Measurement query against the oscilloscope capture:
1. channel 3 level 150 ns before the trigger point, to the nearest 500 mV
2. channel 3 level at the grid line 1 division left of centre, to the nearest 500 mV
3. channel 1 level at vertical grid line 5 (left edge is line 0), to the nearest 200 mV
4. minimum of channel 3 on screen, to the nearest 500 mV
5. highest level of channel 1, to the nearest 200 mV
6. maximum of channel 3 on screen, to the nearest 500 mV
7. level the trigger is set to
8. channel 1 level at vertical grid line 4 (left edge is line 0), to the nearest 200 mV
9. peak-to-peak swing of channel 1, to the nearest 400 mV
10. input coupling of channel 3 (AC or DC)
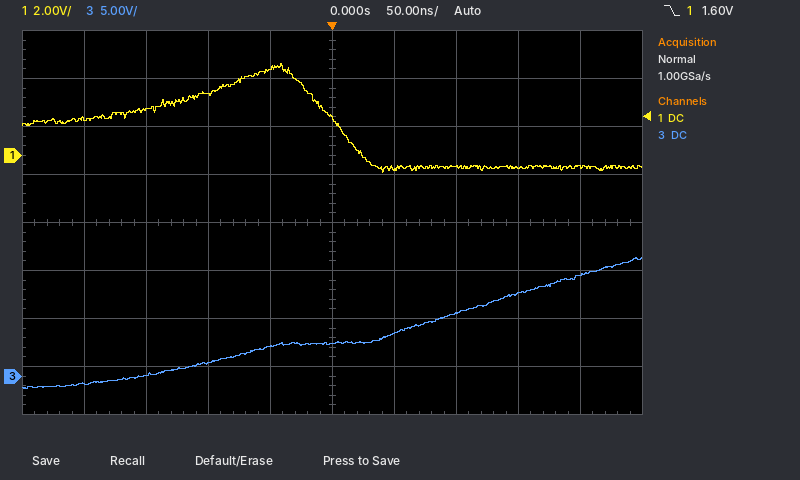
0.0 V
3.0 V
1.6 V
-1.5 V
3.8 V
12.5 V
1.60 V
3.6 V
4.4 V
DC
